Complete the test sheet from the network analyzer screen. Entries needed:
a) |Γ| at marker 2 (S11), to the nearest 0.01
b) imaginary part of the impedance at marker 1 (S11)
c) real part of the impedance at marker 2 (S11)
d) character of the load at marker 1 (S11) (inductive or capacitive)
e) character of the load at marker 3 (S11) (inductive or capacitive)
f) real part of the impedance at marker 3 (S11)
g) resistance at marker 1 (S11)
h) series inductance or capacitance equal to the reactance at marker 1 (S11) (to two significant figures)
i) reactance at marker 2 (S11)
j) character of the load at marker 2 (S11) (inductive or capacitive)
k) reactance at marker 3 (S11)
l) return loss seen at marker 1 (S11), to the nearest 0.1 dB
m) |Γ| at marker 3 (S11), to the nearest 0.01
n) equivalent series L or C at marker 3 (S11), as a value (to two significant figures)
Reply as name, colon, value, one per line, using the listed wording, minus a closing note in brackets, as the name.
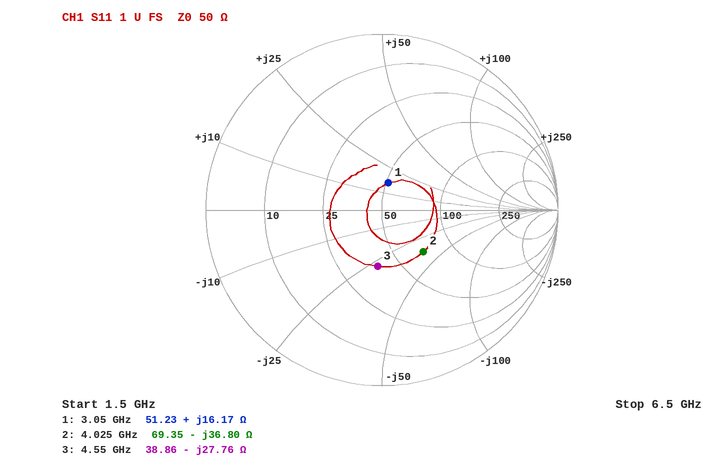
|Γ| at marker 2 (S11), to the nearest 0.01: 0.33
imaginary part of the impedance at marker 1: +16.17 Ω
real part of the impedance at marker 2: 69.35 Ω
character of the load at marker 1 (S11): inductive
character of the load at marker 3 (S11): capacitive
real part of the impedance at marker 3: 38.86 Ω
resistance at marker 1: 51.23 Ω
series inductance or capacitance equal to the reactance at marker 1 (S11): 840 pH
reactance at marker 2: -36.80 Ω
character of the load at marker 2 (S11): capacitive
reactance at marker 3: -27.76 Ω
return loss seen at marker 1 (S11), to the nearest 0.1 dB: 16.0 dB
|Γ| at marker 3 (S11), to the nearest 0.01: 0.32
equivalent series L or C at marker 3 (S11), as a value: 1.3 pF
